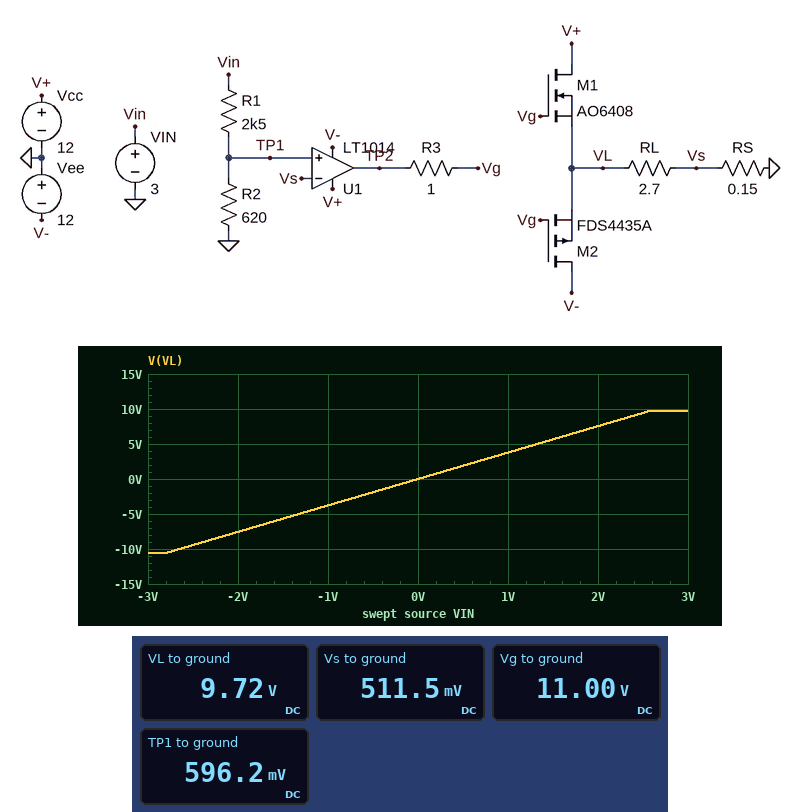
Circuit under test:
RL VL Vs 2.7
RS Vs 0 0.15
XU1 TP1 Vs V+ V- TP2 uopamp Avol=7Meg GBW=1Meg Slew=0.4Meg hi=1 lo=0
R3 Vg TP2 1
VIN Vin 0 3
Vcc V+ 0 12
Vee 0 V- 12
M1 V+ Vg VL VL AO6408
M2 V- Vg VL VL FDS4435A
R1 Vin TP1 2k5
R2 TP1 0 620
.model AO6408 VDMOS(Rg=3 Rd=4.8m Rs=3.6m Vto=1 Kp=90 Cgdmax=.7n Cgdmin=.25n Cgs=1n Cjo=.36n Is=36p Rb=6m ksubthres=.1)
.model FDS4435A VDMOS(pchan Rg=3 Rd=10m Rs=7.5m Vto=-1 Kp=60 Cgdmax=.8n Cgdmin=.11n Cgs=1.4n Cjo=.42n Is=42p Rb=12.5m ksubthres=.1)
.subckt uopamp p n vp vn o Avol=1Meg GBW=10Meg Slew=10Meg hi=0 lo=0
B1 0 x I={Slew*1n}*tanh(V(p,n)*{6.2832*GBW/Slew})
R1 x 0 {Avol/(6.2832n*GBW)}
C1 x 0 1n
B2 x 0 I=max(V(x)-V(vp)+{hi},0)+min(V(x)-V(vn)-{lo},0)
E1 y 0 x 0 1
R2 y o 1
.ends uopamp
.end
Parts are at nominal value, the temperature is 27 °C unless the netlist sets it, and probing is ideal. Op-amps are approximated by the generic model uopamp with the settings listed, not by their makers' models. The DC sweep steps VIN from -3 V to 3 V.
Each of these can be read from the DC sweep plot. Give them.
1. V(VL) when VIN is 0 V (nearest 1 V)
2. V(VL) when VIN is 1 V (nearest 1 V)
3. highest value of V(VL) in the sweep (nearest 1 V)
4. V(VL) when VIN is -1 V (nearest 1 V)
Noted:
0 V
4 V
10 V
-4 V
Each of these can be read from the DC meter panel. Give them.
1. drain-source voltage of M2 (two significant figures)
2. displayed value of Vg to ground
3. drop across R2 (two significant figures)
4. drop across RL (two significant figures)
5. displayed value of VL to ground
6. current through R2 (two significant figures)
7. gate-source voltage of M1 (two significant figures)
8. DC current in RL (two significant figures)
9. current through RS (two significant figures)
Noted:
-22 V
11.00 V
600 mV
9.2 V
9.72 V
960 µA
1.3 V
3.4 A
3.4 A
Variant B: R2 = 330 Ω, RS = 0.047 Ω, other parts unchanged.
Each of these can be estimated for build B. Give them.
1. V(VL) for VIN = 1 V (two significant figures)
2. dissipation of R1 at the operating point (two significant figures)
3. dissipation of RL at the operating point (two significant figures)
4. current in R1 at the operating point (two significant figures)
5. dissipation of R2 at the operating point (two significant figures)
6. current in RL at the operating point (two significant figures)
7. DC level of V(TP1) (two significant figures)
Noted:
6.8 V
2.8 mW
34 W
1.1 mA
370 µW
3.5 A
350 mV
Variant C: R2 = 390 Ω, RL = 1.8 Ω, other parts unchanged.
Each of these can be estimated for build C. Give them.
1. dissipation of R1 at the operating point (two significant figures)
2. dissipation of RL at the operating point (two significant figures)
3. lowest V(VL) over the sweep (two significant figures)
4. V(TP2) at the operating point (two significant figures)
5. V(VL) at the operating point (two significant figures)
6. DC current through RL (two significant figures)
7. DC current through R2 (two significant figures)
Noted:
2.7 mW
13 W
-5.3 V
6.5 V
5.3 V
2.7 A
1.0 mA
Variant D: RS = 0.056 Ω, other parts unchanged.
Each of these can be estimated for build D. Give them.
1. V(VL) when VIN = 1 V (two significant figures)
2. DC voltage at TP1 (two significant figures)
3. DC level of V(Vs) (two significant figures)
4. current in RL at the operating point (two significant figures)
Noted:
9.7 V
600 mV
200 mV
3.5 A
